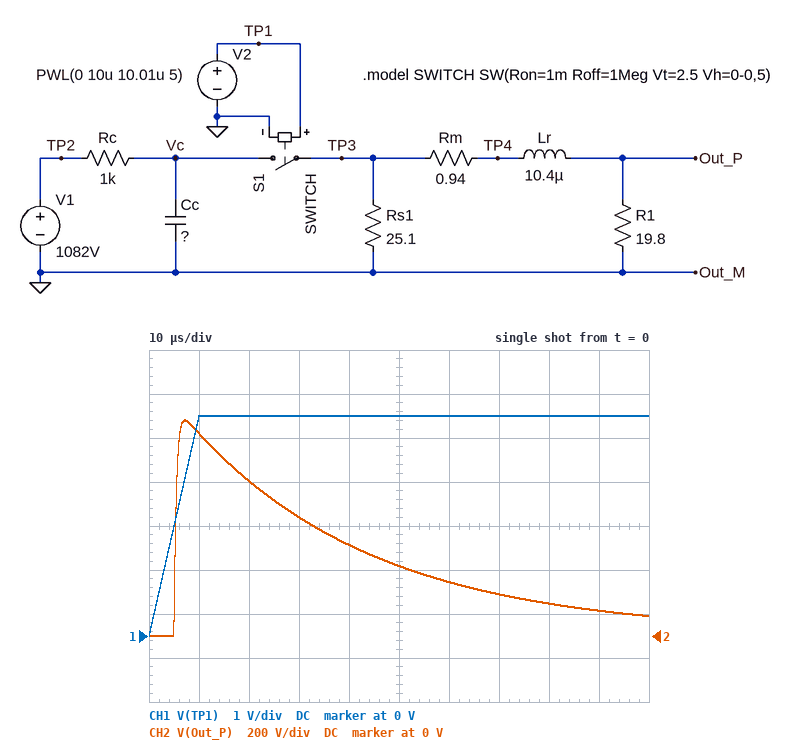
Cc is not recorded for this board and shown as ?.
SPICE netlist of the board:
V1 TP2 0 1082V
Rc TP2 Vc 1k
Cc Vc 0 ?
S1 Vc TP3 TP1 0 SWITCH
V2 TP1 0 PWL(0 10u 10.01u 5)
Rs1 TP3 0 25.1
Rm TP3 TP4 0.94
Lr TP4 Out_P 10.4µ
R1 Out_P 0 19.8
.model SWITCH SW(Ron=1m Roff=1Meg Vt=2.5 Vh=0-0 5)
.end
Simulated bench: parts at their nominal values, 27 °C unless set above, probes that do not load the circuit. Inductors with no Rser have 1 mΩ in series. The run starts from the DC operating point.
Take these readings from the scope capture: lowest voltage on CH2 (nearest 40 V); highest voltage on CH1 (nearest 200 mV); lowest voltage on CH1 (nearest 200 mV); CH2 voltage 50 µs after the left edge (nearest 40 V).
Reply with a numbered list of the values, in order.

1. 0 V
2. 5.0 V
3. 0 V
4. 320 V
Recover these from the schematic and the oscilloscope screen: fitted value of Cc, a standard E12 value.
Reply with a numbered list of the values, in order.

1. 3.3 µF
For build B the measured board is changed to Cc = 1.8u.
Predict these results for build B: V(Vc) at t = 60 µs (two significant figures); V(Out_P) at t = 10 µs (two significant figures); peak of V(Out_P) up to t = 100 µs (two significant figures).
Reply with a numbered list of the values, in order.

1. 81 V
2. 840 V
3. 950 V
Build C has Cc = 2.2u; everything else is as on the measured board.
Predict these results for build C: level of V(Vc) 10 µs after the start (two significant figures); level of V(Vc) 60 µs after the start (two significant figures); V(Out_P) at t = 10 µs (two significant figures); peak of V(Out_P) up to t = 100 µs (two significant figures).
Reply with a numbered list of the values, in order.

1. 890 V
2. 130 V
3. 870 V
4. 960 V
